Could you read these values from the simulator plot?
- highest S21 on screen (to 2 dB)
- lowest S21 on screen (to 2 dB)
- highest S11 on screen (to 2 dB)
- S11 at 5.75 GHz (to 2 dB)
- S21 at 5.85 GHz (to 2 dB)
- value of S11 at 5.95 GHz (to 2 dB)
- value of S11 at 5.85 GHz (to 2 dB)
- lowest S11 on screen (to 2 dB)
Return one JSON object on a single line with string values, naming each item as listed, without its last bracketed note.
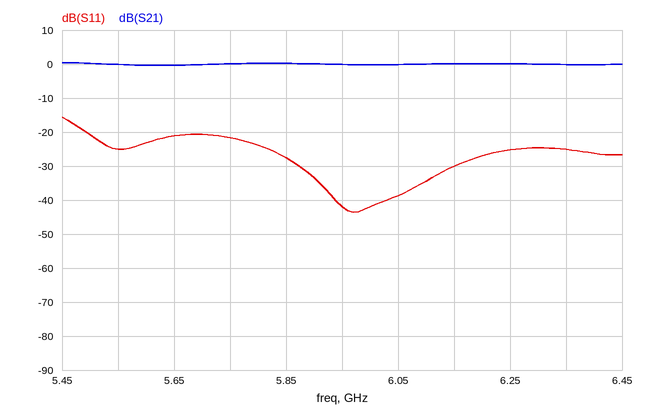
{"highest S21 on screen": "0 dB", "lowest S21 on screen": "0 dB", "highest S11 on screen": "-16 dB", "S11 at 5.75 GHz": "-22 dB", "S21 at 5.85 GHz": "0 dB", "value of S11 at 5.95 GHz": "-42 dB", "value of S11 at 5.85 GHz": "-28 dB", "lowest S11 on screen": "-44 dB"}
